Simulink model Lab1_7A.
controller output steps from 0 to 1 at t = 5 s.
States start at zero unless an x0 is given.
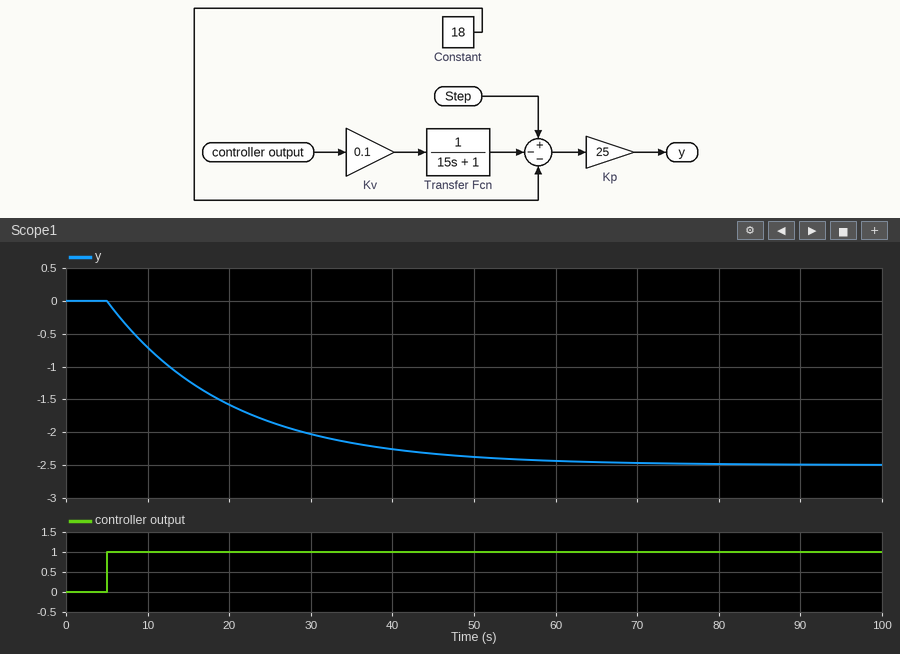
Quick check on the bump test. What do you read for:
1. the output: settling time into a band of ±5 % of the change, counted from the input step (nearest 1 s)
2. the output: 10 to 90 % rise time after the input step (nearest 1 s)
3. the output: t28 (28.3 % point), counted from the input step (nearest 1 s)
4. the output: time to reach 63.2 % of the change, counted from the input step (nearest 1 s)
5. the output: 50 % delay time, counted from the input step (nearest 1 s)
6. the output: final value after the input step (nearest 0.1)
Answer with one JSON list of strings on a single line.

["45 s", "33 s", "5 s", "15 s", "10 s", "-2.5"]
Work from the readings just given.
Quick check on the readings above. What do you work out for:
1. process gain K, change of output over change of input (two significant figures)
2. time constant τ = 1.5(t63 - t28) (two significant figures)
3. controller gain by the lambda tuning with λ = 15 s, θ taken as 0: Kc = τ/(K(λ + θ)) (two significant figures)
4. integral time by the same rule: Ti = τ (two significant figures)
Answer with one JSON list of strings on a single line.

["-2.5", "15 s", "-0.40", "15 s"]
